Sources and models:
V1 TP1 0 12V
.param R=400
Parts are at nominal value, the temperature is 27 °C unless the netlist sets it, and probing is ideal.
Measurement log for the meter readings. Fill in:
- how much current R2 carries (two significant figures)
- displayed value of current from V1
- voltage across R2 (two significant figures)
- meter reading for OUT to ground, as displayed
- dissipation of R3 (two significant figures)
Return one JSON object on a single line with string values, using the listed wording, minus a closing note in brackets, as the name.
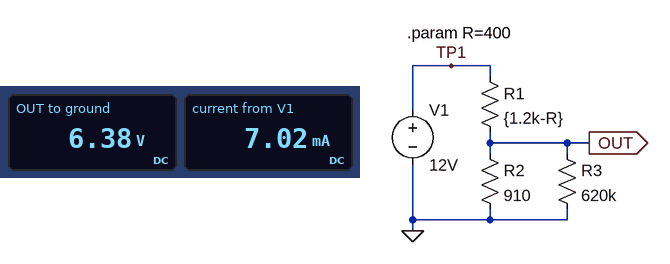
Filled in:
{"how much current R2 carries": "7.0 mA", "displayed value of current from V1": "7.02 mA", "voltage across R2": "6.4 V", "meter reading for OUT to ground, as displayed": "6.38 V", "dissipation of R3": "66 µW"}
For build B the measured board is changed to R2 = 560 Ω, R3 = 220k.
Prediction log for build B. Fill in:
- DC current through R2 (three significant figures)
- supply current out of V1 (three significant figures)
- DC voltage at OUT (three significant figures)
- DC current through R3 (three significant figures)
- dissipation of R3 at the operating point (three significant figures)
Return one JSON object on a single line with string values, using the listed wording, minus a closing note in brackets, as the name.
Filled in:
{"DC current through R2": "8.81 mA", "supply current out of V1": "8.83 mA", "DC voltage at OUT": "4.93 V", "DC current through R3": "22.4 µA", "dissipation of R3 at the operating point": "111 µW"}
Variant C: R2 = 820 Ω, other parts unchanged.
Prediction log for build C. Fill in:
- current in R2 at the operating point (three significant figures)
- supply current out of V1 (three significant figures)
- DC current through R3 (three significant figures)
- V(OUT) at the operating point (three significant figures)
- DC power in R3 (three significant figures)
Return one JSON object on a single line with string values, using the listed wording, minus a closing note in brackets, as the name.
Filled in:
{"current in R2 at the operating point": "7.40 mA", "supply current out of V1": "7.41 mA", "DC current through R3": "9.79 µA", "V(OUT) at the operating point": "6.07 V", "DC power in R3": "59.4 µW"}
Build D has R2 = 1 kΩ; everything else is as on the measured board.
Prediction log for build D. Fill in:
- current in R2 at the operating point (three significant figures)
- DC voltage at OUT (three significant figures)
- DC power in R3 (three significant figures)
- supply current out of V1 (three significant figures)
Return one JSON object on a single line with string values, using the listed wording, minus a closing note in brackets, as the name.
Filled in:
{"current in R2 at the operating point": "6.66 mA", "DC voltage at OUT": "6.66 V", "DC power in R3": "71.6 µW", "supply current out of V1": "6.67 mA"}
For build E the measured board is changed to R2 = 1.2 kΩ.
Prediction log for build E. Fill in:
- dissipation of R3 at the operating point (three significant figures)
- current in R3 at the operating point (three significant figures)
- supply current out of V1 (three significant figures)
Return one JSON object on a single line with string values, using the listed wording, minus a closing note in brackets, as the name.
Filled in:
{"dissipation of R3 at the operating point": "83.5 µW", "current in R3 at the operating point": "11.6 µA", "supply current out of V1": "6.01 mA"}
